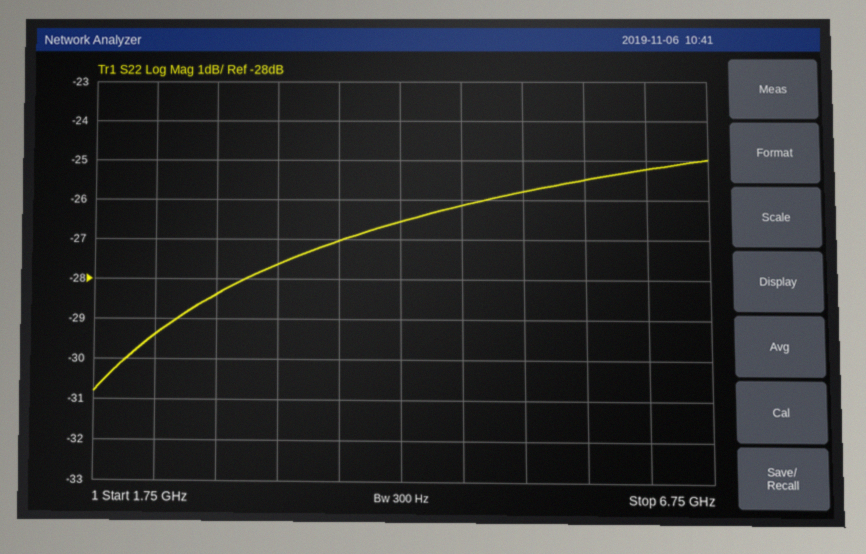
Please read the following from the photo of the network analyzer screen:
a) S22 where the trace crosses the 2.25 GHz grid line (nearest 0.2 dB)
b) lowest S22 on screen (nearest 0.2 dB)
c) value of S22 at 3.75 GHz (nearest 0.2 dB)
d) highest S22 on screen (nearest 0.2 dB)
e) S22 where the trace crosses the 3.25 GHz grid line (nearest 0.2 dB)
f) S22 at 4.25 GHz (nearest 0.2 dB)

-29.4 dB
-30.8 dB
-27.0 dB
-25.0 dB
-27.6 dB
-26.6 dB
